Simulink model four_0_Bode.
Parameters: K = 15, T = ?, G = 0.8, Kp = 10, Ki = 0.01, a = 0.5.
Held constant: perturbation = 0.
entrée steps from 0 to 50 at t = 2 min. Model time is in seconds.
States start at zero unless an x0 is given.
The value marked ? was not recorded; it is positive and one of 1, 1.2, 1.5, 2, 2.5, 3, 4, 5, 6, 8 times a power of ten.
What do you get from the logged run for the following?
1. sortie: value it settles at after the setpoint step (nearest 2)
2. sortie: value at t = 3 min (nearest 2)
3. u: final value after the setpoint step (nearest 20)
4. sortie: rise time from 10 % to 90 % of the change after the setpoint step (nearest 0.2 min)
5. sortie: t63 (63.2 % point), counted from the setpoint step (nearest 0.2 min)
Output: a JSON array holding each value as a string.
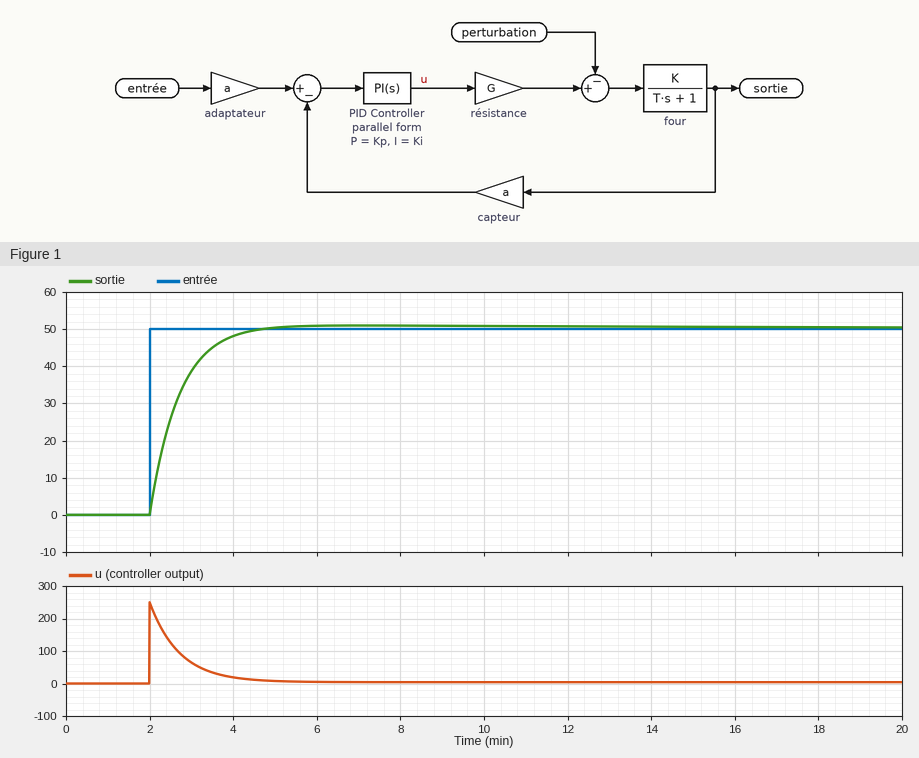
["50", "38", "0", "1.4 min", "0.6 min"]
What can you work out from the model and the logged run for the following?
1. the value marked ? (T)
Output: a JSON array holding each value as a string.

["2500"]
